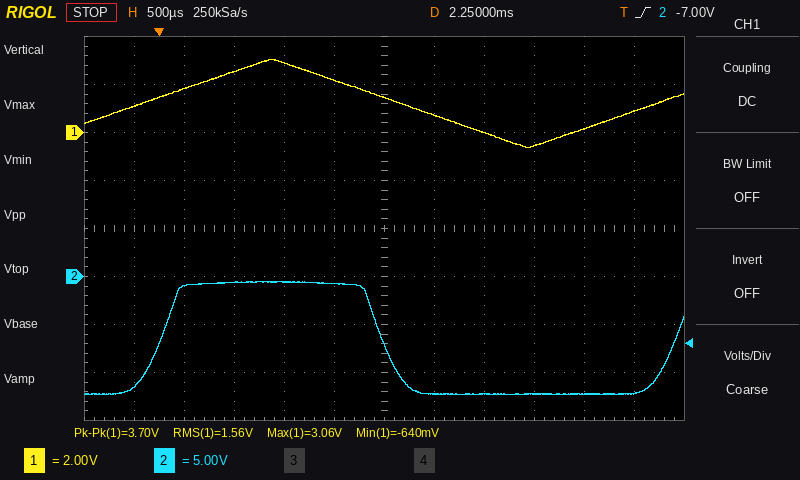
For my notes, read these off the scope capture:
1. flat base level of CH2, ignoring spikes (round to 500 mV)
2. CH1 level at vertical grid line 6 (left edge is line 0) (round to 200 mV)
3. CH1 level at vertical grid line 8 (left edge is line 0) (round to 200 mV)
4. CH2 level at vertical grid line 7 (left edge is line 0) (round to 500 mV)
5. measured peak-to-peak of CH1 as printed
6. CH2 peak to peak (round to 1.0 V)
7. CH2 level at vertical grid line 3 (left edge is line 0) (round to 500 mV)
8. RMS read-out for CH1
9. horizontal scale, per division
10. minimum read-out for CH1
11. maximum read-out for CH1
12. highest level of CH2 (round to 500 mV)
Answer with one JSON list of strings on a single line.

["-12.0 V", "1.4 V", "0.0 V", "-12.0 V", "3.70 V", "12.0 V", "-500 mV", "1.56 V", "500 µs", "-640 mV", "3.06 V", "-500 mV"]
